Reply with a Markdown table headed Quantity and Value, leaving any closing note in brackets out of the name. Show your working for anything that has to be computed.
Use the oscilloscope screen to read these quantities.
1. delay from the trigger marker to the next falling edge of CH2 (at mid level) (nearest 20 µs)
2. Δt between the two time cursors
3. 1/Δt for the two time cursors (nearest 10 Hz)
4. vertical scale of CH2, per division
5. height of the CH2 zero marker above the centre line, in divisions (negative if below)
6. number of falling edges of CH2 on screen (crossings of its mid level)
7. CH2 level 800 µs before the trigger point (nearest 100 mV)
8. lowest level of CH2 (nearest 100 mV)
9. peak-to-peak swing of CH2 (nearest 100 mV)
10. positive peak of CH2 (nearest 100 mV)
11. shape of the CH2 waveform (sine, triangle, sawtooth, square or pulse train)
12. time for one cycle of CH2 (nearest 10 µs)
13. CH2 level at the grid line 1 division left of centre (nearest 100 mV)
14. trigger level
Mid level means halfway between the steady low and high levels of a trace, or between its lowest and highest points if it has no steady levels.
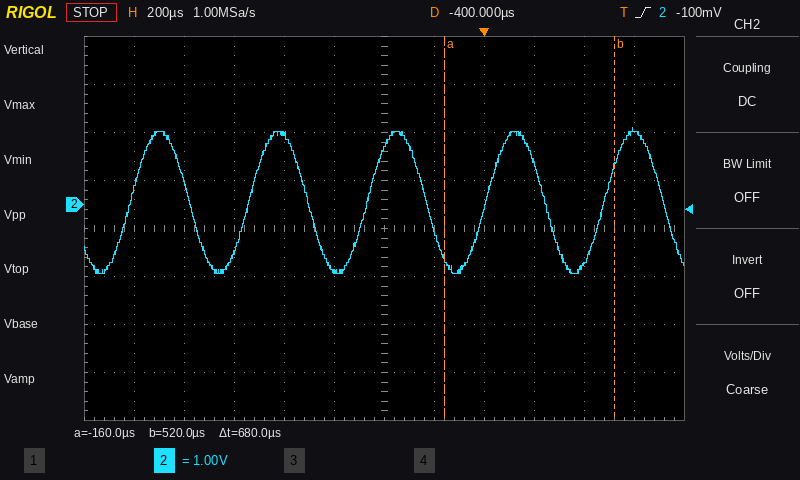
| Quantity | Value |
|---|---|
| delay from the trigger marker to the next falling edge of CH2 (at mid level) | 240 µs |
| Δt between the two time cursors | 680 µs |
| 1/Δt for the two time cursors | 1 / 680 µs ≈ 1.47 kHz |
| vertical scale of CH2, per division | 1 V |
| height of the CH2 zero marker above the centre line, in divisions | +0.5 div |
| number of falling edges of CH2 on screen | 5 |
| CH2 level 800 µs before the trigger point | 1.4 V |
| lowest level of CH2 | -1.4 V |
| peak-to-peak swing of CH2 | 1.6 V − (-1.4 V) = 3.0 V |
| positive peak of CH2 | 1.6 V |
| shape of the CH2 waveform | sine |
| time for one cycle of CH2 | 470 µs |
| CH2 level at the grid line 1 division left of centre | -1.4 V |
| trigger level | -100 mV |
